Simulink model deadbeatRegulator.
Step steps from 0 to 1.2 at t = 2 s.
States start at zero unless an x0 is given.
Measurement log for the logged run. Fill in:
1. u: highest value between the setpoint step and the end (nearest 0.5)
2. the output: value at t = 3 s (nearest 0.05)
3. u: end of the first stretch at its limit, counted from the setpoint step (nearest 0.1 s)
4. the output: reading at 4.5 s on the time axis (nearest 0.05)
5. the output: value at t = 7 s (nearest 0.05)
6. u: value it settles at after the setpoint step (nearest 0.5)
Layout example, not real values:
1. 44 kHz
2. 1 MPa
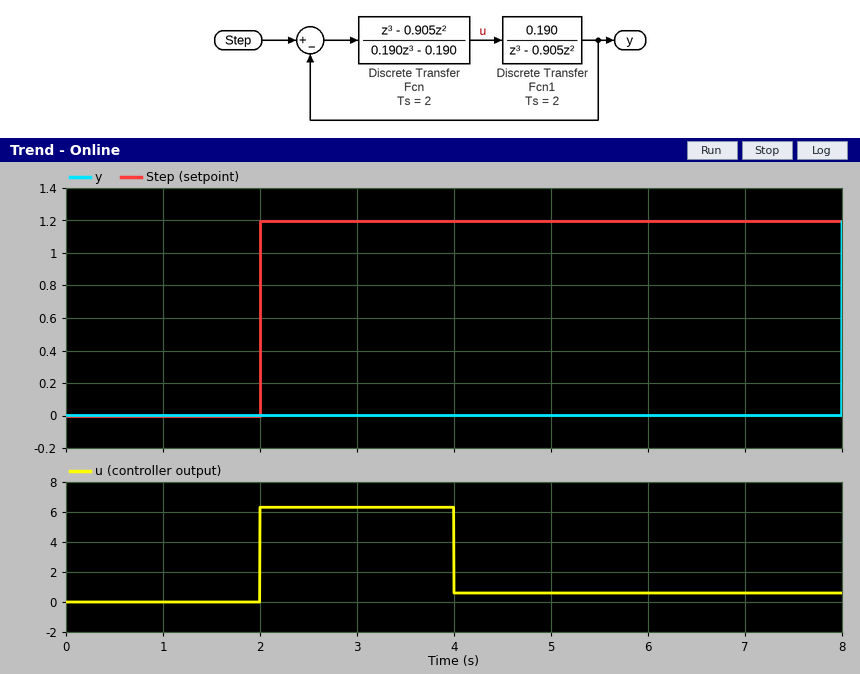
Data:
1. 6.5
2. 0.00
3. 2.0 s
4. 0.00
5. 0.00
6. 0.5
